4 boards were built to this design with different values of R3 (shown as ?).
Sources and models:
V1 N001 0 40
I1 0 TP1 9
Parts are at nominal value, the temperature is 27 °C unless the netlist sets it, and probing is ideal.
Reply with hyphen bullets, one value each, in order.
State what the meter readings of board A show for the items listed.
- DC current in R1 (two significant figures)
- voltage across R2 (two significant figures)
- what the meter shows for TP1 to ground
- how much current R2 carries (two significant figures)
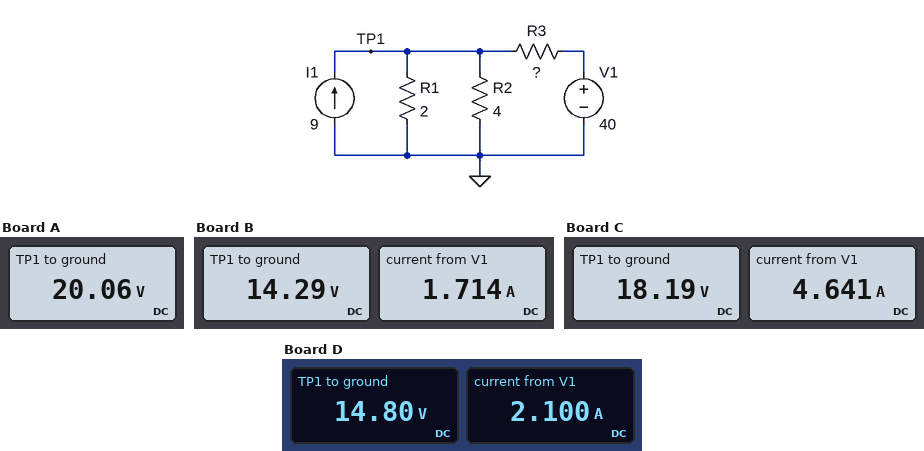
- 10 A
- 20 V
- 20.06 V
- 5.0 A
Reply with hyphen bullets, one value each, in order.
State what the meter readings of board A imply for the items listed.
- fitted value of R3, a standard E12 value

- 3.3 Ω
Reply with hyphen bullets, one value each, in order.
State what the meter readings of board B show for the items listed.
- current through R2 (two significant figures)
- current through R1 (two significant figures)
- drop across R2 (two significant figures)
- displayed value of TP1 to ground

- 3.6 A
- 7.1 A
- 14 V
- 14.29 V
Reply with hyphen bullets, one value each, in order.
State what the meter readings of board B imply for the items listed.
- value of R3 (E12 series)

- 15 Ω
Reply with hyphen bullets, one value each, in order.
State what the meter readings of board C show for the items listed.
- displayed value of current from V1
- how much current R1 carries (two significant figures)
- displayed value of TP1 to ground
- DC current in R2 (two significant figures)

- 4.641 A
- 9.1 A
- 18.19 V
- 4.5 A
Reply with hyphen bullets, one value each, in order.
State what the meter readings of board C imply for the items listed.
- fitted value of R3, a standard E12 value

- 4.7 Ω
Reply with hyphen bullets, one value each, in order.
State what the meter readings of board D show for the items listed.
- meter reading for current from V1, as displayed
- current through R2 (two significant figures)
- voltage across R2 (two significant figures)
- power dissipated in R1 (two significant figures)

- 2.100 A
- 3.7 A
- 15 V
- 110 W
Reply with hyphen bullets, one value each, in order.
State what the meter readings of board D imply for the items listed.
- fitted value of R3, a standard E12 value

- 12 Ω
